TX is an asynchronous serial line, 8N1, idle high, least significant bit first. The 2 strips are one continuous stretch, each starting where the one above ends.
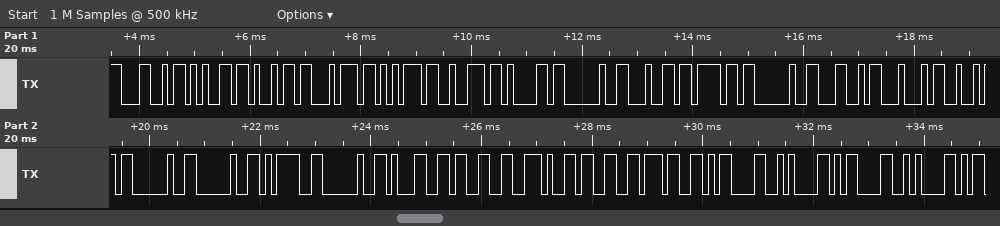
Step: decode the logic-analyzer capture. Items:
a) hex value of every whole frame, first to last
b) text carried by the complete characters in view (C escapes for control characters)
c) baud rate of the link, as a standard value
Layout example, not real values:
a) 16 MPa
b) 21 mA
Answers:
a) 4C 65 69 74 75 72 61 20 64 6F 20 4C 44 52 20 20 3D 20 31 33 2E 33 37 0D 0A 0D 0A
b) "Leitura do LDR  = 13.37\r\n\r\n"
c) 9600 baud
